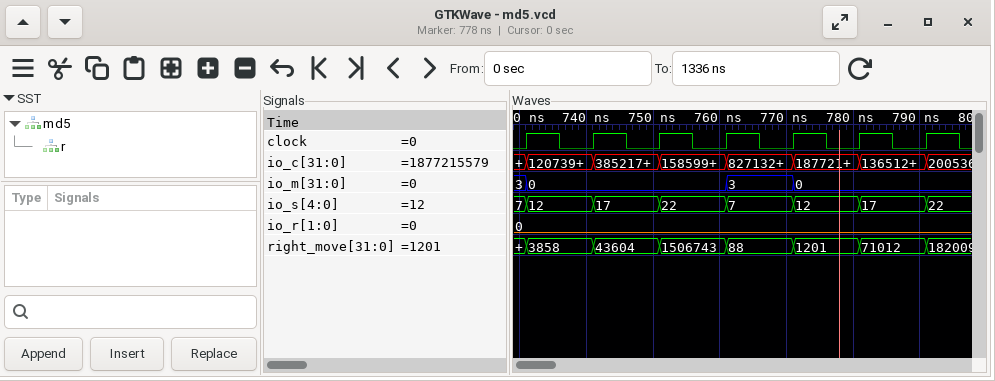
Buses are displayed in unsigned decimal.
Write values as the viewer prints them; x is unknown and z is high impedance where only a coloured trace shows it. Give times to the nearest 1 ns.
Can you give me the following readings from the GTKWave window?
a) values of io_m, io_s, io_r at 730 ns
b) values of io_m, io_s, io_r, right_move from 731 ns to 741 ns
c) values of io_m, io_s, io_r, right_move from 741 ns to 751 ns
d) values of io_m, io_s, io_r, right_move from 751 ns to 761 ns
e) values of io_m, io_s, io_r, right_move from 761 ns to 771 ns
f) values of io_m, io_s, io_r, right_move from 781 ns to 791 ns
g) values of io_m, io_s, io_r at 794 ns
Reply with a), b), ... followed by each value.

a) io_m=3, io_s=7, io_r=0
b) io_m=0, io_s=12, io_r=0, right_move=3858
c) io_m=0, io_s=17, io_r=0, right_move=43604
d) io_m=0, io_s=22, io_r=0, right_move=1506743
e) io_m=3, io_s=7, io_r=0, right_move=88
f) io_m=0, io_s=17, io_r=0, right_move=71012
g) io_m=0, io_s=22, io_r=0
